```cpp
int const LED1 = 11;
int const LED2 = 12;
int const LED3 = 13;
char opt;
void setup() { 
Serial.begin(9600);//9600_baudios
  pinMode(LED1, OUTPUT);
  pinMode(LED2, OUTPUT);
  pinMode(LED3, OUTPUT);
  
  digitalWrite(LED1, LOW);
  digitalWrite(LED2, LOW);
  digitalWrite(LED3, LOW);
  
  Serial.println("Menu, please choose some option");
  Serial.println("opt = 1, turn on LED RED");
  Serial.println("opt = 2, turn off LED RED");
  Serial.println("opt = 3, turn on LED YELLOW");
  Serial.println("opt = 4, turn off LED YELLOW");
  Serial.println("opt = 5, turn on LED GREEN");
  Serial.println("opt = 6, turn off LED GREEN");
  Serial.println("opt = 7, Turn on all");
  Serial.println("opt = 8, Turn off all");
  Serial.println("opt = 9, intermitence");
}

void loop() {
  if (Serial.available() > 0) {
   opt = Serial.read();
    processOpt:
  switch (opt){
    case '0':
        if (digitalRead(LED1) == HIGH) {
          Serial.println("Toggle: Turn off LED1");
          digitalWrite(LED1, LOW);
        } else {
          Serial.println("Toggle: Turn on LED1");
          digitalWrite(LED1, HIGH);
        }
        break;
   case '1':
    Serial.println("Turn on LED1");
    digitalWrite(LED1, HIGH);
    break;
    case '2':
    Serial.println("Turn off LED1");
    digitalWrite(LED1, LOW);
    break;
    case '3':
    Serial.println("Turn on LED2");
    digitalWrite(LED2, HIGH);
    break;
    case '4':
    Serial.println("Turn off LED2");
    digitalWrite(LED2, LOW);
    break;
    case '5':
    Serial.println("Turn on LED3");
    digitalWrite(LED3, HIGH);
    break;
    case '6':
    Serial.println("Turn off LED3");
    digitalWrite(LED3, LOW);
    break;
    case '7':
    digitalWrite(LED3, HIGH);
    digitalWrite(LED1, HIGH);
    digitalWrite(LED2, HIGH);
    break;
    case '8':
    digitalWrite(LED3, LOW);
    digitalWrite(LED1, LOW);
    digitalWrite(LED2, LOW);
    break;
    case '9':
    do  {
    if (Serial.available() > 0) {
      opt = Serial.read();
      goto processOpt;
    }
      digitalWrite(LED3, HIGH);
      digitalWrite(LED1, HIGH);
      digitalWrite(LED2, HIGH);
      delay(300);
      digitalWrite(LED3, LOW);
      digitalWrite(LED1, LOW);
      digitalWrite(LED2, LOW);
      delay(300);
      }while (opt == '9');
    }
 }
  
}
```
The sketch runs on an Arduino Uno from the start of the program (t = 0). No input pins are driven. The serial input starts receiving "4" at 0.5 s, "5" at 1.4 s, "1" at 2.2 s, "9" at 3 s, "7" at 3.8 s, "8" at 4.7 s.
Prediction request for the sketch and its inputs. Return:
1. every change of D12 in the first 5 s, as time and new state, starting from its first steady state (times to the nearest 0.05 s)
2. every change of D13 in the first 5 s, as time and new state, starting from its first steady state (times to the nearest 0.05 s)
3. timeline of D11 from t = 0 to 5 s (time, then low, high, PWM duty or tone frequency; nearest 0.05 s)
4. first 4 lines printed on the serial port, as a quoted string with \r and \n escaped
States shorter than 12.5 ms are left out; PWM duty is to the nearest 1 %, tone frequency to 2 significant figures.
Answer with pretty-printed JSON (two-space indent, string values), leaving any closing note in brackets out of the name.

{
  "every change of D12 in the first 5 s, as time and new state, starting from its first steady state": "0 s low; 3 s high; 3.3 s low; 3.6 s high; 3.9 s low; 4.2 s high; 4.7 s low",
  "every change of D13 in the first 5 s, as time and new state, starting from its first steady state": "0 s low; 1.4 s high; 3.3 s low; 3.6 s high; 3.9 s low; 4.2 s high; 4.7 s low",
  "timeline of D11 from t = 0 to 5 s": "0 s low; 2.2 s high; 3.3 s low; 3.6 s high; 3.9 s low; 4.2 s high; 4.7 s low",
  "first 4 lines printed on the serial port, as a quoted string with \\r and \\n escaped": "\"Menu, please choose some option\\r\\nopt = 1, turn on LED RED\\r\\nopt = 2, turn off LED RED\\r\\nopt = 3, turn on LED YELLOW\\r\\n\""
}
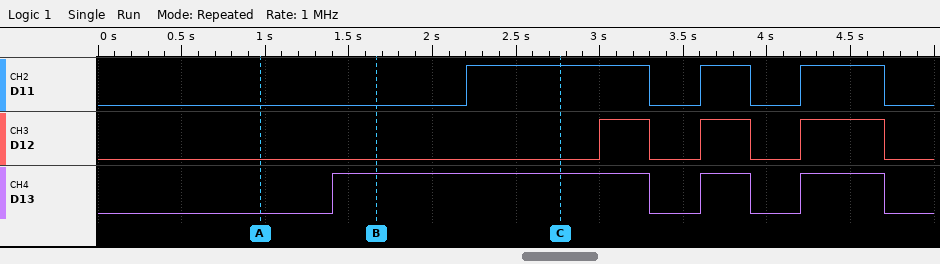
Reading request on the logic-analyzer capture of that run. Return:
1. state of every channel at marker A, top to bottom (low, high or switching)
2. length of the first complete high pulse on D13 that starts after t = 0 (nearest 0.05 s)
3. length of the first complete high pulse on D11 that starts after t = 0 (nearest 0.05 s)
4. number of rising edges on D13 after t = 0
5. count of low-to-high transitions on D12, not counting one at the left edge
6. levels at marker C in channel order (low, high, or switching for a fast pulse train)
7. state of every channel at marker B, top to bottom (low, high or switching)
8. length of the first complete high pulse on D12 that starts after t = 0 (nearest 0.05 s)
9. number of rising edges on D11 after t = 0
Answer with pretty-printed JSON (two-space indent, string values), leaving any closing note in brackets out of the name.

{
  "state of every channel at marker A, top to bottom": "D11 low, D12 low, D13 low",
  "length of the first complete high pulse on D13 that starts after t = 0": "1.90 s",
  "length of the first complete high pulse on D11 that starts after t = 0": "1.10 s",
  "number of rising edges on D13 after t = 0": "3",
  "count of low-to-high transitions on D12, not counting one at the left edge": "3",
  "levels at marker C in channel order": "D11 high, D12 low, D13 high",
  "state of every channel at marker B, top to bottom": "D11 low, D12 low, D13 high",
  "length of the first complete high pulse on D12 that starts after t = 0": "0.30 s",
  "number of rising edges on D11 after t = 0": "3"
}
